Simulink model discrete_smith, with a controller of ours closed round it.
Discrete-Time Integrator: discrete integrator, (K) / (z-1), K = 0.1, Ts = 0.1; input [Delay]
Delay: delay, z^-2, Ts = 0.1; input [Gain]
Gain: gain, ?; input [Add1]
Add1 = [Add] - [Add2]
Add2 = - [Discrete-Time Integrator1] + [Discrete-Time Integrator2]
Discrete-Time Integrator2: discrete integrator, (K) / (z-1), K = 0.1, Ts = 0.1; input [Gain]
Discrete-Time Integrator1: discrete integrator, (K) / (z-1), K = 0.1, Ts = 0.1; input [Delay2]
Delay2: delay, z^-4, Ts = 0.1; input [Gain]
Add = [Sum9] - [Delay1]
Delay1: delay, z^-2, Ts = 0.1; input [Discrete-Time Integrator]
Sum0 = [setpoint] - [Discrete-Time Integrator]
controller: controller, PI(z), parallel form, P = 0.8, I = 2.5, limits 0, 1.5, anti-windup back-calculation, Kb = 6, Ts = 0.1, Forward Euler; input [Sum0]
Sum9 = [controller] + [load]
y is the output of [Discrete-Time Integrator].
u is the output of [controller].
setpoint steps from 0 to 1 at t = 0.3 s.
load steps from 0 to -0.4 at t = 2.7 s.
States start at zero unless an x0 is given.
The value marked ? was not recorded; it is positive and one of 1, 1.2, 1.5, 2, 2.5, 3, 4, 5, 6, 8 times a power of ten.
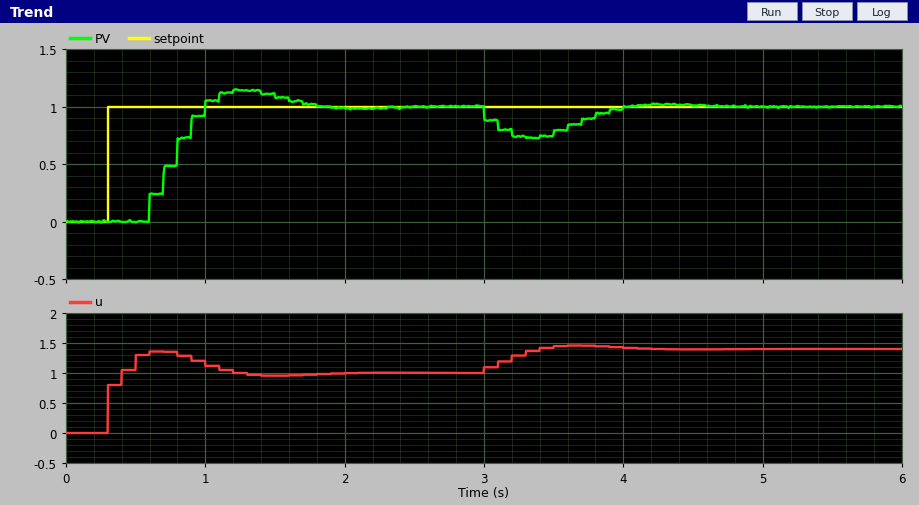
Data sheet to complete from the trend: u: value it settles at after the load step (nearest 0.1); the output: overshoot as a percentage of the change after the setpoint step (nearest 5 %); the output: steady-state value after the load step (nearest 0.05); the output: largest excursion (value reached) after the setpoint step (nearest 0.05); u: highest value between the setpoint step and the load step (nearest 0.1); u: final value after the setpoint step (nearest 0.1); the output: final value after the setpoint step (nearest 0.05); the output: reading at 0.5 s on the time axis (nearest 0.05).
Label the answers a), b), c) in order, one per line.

a) 1.4
b) 15 %
c) 1.00
d) 1.15
e) 1.4
f) 1.0
g) 1.00
h) 0.00
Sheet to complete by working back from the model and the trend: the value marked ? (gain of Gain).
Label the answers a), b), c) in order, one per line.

a) 3
